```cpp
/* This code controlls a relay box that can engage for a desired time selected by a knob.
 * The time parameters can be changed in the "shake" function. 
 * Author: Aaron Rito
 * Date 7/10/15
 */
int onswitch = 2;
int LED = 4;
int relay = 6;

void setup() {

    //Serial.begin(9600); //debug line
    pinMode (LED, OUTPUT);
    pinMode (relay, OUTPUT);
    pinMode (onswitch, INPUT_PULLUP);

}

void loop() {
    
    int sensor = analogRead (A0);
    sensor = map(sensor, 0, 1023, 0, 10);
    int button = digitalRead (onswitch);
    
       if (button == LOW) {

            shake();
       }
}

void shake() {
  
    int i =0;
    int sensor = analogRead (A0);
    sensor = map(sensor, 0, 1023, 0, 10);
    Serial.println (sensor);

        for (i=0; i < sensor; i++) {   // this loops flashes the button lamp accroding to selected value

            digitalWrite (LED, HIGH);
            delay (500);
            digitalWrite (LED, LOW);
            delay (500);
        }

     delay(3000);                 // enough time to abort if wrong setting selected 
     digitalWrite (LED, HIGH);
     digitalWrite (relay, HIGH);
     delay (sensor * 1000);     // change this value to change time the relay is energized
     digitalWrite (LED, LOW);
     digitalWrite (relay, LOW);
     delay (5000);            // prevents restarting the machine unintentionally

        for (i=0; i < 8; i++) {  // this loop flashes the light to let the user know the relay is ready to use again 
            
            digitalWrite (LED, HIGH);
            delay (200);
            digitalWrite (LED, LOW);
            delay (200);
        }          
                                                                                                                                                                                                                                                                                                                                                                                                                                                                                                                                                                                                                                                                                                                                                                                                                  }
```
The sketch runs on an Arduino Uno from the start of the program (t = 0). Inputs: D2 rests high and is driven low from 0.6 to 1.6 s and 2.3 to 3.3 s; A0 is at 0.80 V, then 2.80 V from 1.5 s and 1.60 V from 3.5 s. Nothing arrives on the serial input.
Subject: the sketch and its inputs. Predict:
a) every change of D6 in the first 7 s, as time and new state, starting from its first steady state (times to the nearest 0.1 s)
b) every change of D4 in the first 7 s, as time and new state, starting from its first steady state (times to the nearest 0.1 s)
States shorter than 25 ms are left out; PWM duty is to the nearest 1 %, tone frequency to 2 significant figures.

0 s low; 4.6 s high; 5.6 s low
0 s low; 0.6 s high; 1.1 s low; 4.6 s high; 5.6 s low
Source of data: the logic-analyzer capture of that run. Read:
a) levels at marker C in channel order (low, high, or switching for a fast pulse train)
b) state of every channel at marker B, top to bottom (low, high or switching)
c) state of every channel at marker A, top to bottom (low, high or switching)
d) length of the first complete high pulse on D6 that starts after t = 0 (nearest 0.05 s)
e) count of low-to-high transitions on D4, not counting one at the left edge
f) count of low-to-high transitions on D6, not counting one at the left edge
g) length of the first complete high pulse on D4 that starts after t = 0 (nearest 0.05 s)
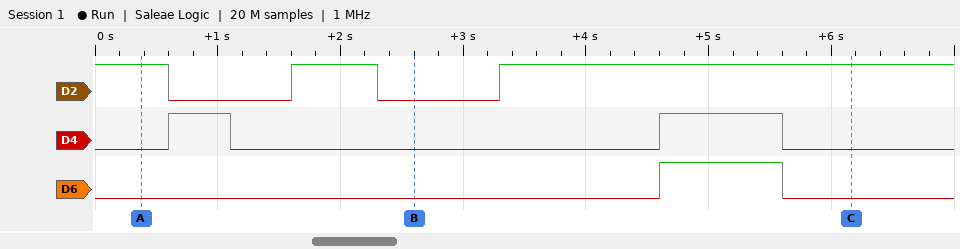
D2 high, D4 low, D6 low
D2 low, D4 low, D6 low
D2 high, D4 low, D6 low
1.00 s
2
1
0.50 s
